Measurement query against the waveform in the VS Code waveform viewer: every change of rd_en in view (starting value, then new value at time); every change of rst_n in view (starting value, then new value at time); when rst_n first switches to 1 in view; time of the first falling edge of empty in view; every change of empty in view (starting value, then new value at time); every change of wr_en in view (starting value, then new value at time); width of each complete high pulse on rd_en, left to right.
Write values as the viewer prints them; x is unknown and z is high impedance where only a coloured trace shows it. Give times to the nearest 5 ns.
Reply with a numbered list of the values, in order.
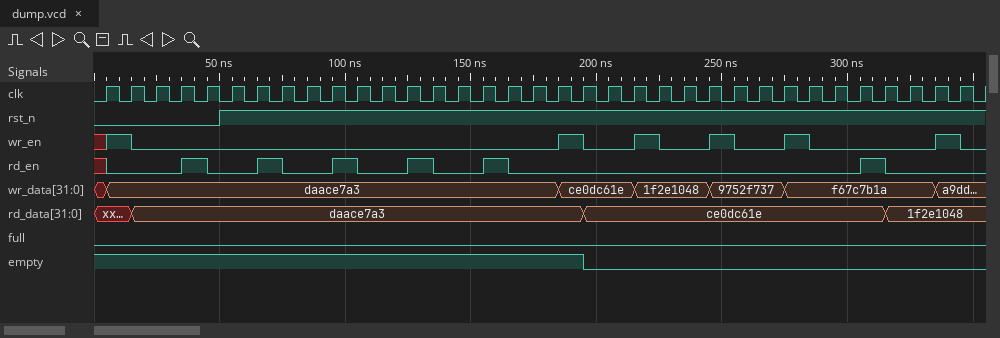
1. x, 0 at 5 ns, 1 at 35 ns, 0 at 45 ns, 1 at 65 ns, 0 at 75 ns, 1 at 95 ns, 0 at 105 ns, 1 at 125 ns, 0 at 135 ns, 1 at 155 ns, 0 at 165 ns, 1 at 305 ns, 0 at 315 ns
2. 0, 1 at 50 ns
3. 50 ns
4. 195 ns
5. 1, 0 at 195 ns
6. x, 1 at 5 ns, 0 at 15 ns, 1 at 185 ns, 0 at 195 ns, 1 at 215 ns, 0 at 225 ns, 1 at 245 ns, 0 at 255 ns, 1 at 275 ns, 0 at 285 ns, 1 at 335 ns, 0 at 345 ns
7. 10 ns, 10 ns, 10 ns, 10 ns, 10 ns, 10 ns
